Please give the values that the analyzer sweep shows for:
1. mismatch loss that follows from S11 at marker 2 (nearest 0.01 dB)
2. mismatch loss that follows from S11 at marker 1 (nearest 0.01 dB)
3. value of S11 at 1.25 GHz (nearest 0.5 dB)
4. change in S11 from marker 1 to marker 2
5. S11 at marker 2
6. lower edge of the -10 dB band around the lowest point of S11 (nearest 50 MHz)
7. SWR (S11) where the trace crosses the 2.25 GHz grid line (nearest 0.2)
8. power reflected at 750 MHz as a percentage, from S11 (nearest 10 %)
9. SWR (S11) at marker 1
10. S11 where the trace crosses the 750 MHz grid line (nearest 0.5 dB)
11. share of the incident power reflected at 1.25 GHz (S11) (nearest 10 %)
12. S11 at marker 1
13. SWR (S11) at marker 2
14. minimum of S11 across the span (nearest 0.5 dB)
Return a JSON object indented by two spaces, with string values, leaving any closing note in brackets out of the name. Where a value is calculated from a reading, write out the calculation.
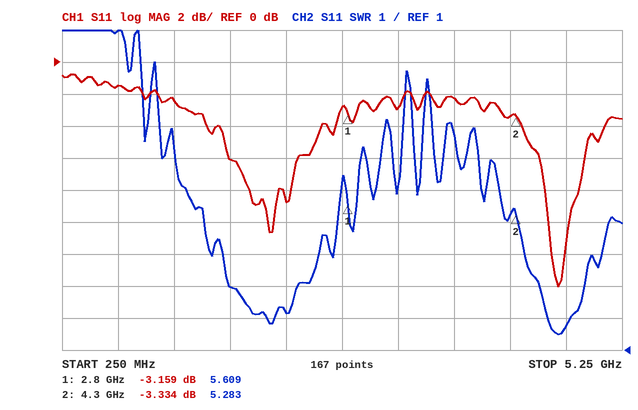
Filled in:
{
  "mismatch loss that follows from S11 at marker 2": "−10 log10(1 − 10^(-3.334/10)) ≈ 2.71 dB",
  "mismatch loss that follows from S11 at marker 1": "−10 log10(1 − 10^(-3.159/10)) ≈ 2.87 dB",
  "value of S11 at 1.25 GHz": "-2.5 dB",
  "change in S11 from marker 1 to marker 2": "-3.334 − (-3.159) = -0.175 dB",
  "S11 at marker 2": "-3.334 dB",
  "lower edge of the -10 dB band around the lowest point of S11": "4.60 GHz",
  "SWR (S11) where the trace crosses the 2.25 GHz grid line": "2.2",
  "power reflected at 750 MHz as a percentage, from S11": "10^(-1.5/10) ≈ 70.8 %, so 70 % to the nearest 10 %",
  "SWR (S11) at marker 1": "5.609",
  "S11 where the trace crosses the 750 MHz grid line": "-1.5 dB",
  "share of the incident power reflected at 1.25 GHz (S11)": "10^(-2.5/10) ≈ 56.2 %, so 60 % to the nearest 10 %",
  "S11 at marker 1": "-3.159 dB",
  "SWR (S11) at marker 2": "5.283",
  "minimum of S11 across the span": "-14.0 dB"
}
